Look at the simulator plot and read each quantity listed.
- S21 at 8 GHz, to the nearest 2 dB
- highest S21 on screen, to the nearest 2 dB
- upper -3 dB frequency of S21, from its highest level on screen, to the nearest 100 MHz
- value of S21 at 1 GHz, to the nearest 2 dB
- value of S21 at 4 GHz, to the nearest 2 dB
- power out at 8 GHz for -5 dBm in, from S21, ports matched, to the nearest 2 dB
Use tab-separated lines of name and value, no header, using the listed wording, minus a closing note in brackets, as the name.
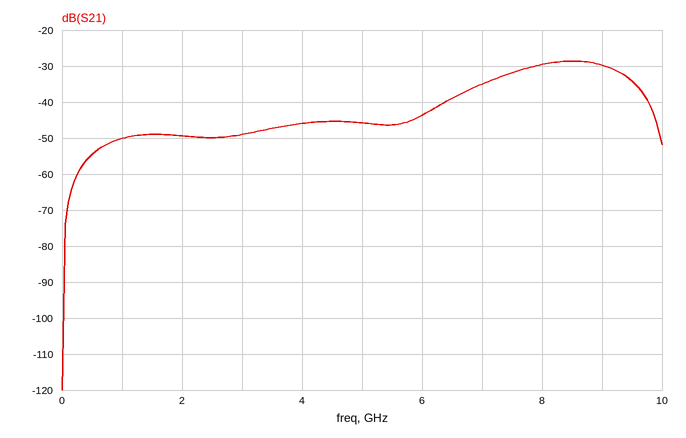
S21 at 8 GHz, to the nearest 2 dB	-30 dB
highest S21 on screen, to the nearest 2 dB	-28 dB
upper -3 dB frequency of S21, from its highest level on screen, to the nearest 100 MHz	9.3 GHz
value of S21 at 1 GHz, to the nearest 2 dB	-50 dB
value of S21 at 4 GHz, to the nearest 2 dB	-46 dB
power out at 8 GHz for -5 dBm in, from S21, ports matched, to the nearest 2 dB	-34 dBm
